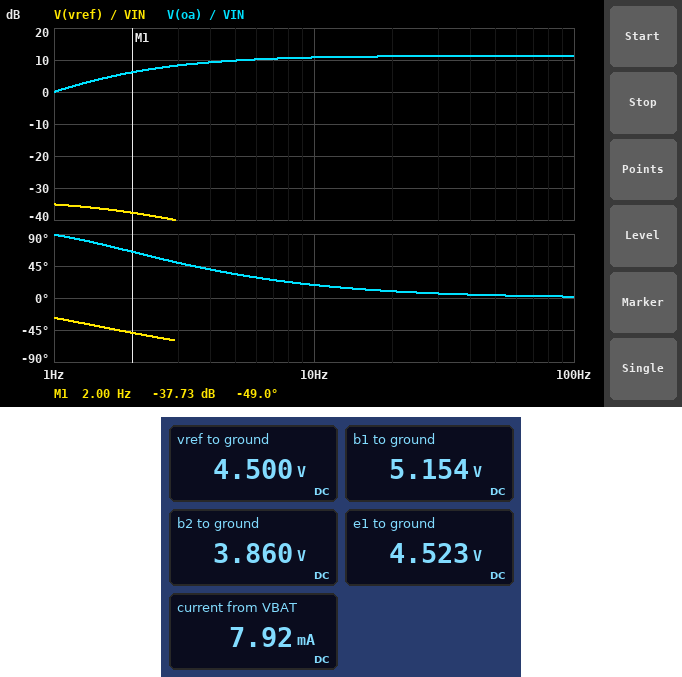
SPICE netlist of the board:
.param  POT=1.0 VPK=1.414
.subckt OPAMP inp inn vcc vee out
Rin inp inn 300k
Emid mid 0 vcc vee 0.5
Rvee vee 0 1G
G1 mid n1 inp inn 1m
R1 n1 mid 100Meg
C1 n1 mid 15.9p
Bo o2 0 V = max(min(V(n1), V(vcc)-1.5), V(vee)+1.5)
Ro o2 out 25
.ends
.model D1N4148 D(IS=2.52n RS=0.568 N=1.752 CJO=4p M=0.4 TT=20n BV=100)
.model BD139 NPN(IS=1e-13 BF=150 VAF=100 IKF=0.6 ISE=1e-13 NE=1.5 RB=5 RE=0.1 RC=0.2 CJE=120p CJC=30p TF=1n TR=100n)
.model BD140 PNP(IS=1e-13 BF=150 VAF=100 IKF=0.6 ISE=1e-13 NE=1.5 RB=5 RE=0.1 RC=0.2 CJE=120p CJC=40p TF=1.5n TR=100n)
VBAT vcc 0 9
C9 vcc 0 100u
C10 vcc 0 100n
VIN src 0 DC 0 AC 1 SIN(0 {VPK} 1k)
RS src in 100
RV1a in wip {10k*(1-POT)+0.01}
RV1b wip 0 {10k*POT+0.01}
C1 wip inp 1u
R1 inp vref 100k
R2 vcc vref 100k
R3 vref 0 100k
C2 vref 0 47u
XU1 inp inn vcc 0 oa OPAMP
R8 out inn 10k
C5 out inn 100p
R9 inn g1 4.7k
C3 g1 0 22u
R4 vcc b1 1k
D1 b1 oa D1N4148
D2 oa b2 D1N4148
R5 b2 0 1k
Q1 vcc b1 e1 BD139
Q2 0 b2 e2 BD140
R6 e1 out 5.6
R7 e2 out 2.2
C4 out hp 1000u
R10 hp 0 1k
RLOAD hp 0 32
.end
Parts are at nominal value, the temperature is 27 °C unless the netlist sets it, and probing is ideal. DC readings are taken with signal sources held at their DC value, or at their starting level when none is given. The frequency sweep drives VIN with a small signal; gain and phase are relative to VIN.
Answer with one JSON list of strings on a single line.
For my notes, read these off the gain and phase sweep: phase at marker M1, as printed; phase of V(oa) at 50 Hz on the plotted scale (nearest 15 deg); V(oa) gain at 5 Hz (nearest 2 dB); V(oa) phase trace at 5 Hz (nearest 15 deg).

["-49.0 deg", "0 deg", "10 dB", "30 deg"]
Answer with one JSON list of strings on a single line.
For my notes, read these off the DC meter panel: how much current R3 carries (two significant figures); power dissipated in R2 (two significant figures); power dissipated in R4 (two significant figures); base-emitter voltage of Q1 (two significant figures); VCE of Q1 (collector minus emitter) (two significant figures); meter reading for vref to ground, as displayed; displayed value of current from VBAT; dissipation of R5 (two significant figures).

["45 µA", "200 µW", "15 mW", "630 mV", "4.5 V", "4.500 V", "7.92 mA", "15 mW"]
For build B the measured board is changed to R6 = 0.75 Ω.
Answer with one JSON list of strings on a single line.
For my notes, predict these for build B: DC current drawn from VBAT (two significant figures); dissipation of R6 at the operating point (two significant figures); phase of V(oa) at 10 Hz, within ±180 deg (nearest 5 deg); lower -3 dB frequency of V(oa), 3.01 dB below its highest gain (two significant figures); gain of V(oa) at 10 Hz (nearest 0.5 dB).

["9.3 mA", "22 µW", "15 deg", "2.7 Hz", "10.5 dB"]
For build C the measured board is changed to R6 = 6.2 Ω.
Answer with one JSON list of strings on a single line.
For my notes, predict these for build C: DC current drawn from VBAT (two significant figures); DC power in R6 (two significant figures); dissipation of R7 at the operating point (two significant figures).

["7.8 mA", "96 µW", "34 µW"]
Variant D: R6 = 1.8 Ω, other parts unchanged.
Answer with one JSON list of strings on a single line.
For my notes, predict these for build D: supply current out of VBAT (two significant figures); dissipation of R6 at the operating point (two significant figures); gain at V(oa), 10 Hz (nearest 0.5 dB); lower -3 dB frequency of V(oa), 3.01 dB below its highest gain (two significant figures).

["8.9 mA", "45 µW", "10.5 dB", "2.8 Hz"]
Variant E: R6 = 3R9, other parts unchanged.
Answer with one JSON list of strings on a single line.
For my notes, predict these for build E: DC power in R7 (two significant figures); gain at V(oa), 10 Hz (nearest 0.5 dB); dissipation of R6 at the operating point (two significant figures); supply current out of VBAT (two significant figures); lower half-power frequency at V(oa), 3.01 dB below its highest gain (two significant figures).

["43 µW", "10.5 dB", "76 µW", "8.3 mA", "2.9 Hz"]
